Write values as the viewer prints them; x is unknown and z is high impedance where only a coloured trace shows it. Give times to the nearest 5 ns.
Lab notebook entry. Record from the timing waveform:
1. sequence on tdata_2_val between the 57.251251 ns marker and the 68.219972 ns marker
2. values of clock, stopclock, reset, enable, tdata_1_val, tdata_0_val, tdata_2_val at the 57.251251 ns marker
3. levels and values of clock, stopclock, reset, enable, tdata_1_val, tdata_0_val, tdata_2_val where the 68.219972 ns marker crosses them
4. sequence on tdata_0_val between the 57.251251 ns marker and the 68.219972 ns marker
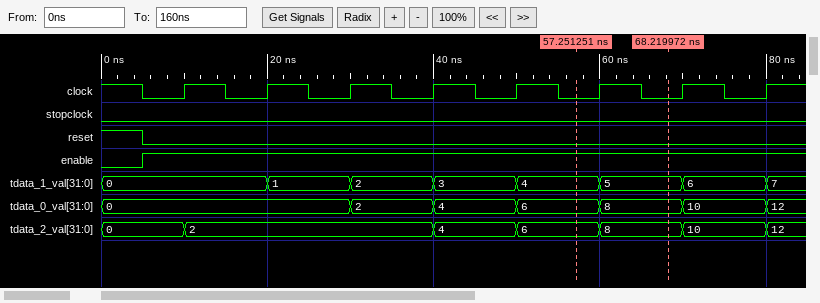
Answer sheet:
6, 8
clock=0, stopclock=0, reset=0, enable=1, tdata_1_val=4, tdata_0_val=6, tdata_2_val=6
clock=0, stopclock=0, reset=0, enable=1, tdata_1_val=5, tdata_0_val=8, tdata_2_val=8
6, 8
